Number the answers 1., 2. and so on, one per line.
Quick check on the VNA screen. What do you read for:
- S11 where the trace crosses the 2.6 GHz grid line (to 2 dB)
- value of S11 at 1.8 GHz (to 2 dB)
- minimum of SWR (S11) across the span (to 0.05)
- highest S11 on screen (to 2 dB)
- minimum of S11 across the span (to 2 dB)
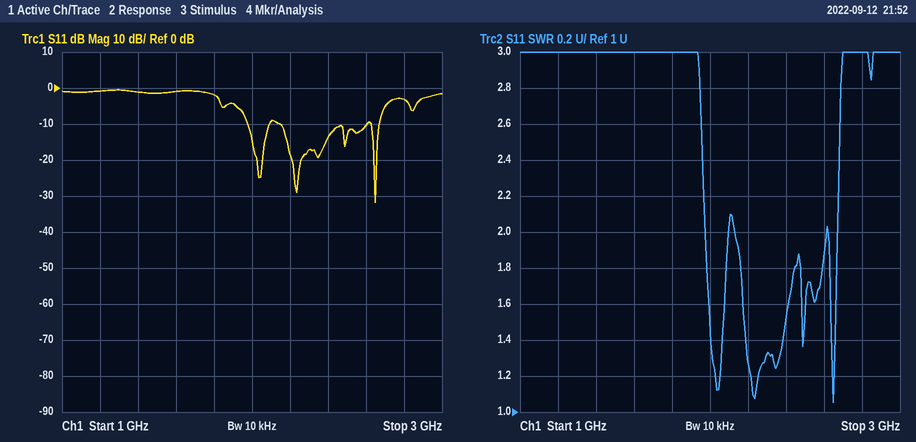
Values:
1. -10 dB
2. -2 dB
3. 1.05
4. 0 dB
5. -32 dB
